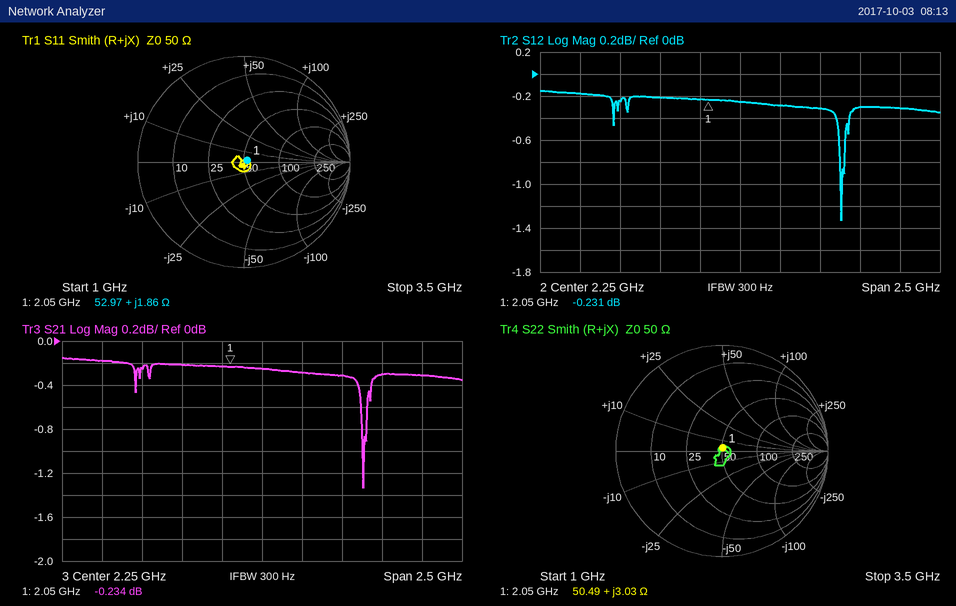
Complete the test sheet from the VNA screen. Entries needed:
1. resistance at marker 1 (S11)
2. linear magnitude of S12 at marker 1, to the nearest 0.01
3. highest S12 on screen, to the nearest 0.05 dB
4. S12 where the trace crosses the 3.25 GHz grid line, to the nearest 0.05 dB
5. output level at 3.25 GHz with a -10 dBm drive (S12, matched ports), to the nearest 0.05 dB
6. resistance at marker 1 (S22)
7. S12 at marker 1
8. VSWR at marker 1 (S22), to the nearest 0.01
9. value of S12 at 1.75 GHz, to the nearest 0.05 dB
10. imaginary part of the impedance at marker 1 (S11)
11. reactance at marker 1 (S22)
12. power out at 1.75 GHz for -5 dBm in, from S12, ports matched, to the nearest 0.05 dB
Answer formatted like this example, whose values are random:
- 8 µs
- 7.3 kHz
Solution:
- 52.97 Ω
- 0.97
- -0.15 dB
- -0.30 dB
- -10.30 dBm
- 50.49 Ω
- -0.231 dB
- 1.06
- -0.20 dB
- +1.86 Ω
- +3.03 Ω
- -5.20 dBm
